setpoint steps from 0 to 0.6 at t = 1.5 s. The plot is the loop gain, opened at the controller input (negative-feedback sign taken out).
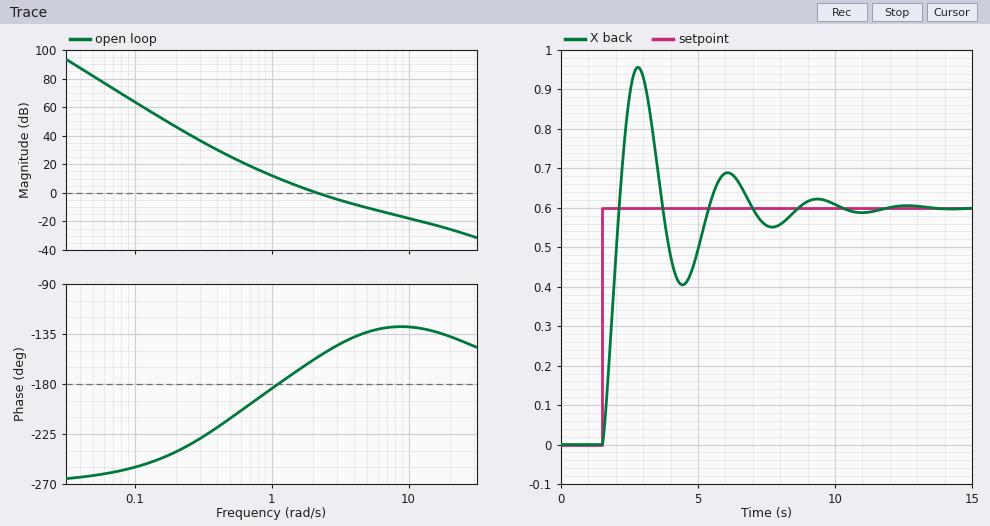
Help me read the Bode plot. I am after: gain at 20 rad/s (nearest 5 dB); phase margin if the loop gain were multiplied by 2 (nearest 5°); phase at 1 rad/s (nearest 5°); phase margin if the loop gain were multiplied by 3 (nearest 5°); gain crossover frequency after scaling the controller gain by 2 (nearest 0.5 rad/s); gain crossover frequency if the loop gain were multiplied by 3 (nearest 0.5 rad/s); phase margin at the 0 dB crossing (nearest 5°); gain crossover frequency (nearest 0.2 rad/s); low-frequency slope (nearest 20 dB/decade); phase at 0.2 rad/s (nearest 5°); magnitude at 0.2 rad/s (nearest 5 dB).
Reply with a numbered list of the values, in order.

1. -25 dB
2. 40°
3. -185°
4. 45°
5. 3.5 rad/s
6. 4.5 rad/s
7. 25°
8. 2.2 rad/s
9. -60 dB/decade
10. -240°
11. 45 dB
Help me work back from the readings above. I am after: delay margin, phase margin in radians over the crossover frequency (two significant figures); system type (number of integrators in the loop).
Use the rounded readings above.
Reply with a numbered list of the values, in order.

1. 0.20 s
2. 3
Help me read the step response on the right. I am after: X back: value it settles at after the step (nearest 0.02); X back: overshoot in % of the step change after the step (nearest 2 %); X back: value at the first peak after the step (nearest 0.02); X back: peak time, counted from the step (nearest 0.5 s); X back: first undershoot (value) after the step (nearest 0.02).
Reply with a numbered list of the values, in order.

1. 0.60
2. 60 %
3. 0.96
4. 1.5 s
5. 0.40
